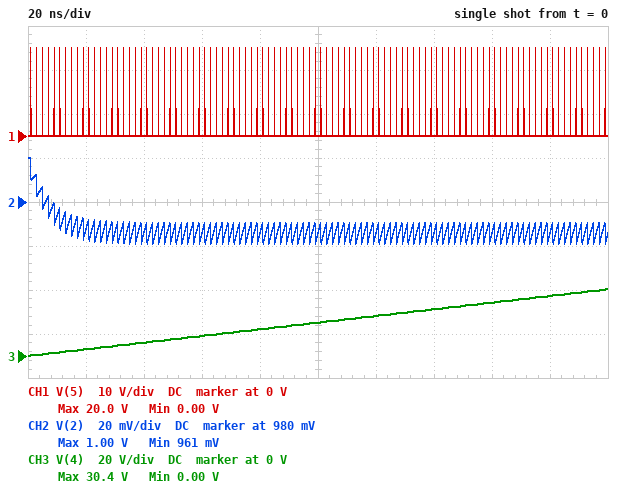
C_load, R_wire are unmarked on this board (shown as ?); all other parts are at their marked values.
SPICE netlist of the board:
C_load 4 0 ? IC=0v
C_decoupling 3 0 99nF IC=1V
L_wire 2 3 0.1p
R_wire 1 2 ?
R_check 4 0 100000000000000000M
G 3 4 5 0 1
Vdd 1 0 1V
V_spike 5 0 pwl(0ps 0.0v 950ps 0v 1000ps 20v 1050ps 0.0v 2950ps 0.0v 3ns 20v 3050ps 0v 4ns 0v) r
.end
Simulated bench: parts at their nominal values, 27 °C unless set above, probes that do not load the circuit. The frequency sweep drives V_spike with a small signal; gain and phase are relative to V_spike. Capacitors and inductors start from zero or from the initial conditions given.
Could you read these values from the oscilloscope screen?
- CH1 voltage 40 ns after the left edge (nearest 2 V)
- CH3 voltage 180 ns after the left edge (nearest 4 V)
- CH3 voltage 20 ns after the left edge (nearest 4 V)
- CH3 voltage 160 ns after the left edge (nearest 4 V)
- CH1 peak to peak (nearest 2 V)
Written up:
0 V
28 V
4 V
24 V
20 V
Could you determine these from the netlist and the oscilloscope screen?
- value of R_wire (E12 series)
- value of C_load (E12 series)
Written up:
0.068 Ω
3.3 nF
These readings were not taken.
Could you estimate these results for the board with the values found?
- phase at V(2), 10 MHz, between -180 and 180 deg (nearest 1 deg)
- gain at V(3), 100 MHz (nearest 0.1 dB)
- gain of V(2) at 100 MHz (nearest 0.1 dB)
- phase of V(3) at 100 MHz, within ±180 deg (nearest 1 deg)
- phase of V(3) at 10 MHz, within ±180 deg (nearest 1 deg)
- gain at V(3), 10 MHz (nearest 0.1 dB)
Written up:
157 deg
-36.1 dB
-36.1 dB
103 deg
157 deg
-24.1 dB
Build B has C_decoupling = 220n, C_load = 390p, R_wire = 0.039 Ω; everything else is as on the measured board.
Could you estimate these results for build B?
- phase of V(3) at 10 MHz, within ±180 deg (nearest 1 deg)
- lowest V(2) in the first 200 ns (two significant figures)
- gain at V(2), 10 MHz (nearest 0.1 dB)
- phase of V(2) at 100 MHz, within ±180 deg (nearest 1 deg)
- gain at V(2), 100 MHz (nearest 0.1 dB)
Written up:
152 deg
980 mV
-29.3 dB
100 deg
-43.0 dB
